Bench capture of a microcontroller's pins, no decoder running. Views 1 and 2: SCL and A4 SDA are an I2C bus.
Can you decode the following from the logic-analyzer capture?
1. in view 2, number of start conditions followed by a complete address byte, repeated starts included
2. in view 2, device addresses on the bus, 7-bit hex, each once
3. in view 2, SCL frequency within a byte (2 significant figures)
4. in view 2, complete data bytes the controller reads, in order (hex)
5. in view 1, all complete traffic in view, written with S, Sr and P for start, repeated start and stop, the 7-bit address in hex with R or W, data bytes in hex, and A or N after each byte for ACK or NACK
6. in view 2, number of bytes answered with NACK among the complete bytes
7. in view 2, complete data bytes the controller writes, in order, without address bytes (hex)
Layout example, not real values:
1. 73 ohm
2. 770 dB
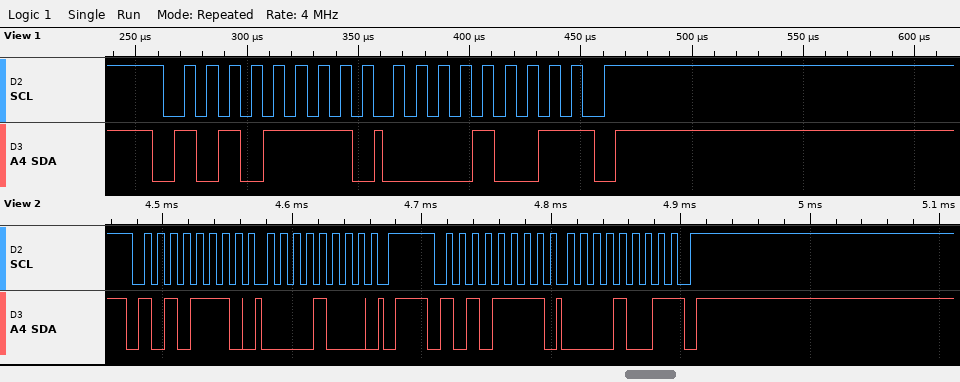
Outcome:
1. 2
2. 0x57
3. 100 kHz
4. 09
5. S 57R A 09 N P
6. 1
7. 08
